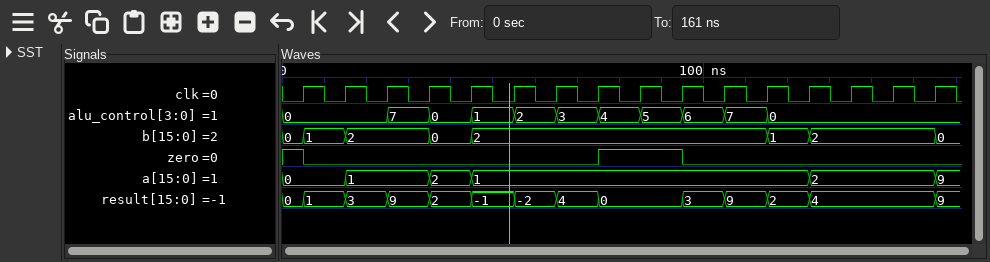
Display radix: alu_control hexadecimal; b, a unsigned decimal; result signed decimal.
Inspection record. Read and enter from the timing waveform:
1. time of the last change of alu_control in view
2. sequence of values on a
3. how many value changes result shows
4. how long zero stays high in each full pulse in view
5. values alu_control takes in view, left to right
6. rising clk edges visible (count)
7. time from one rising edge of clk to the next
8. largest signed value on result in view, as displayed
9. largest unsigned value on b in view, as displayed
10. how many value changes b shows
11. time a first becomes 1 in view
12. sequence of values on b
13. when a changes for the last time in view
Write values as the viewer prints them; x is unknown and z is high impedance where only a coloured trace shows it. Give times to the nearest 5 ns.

115 ns
0, 1, 2, 1, 2, 9
13
20 ns
0, 7, 0, 1, 2, 3, 4, 5, 6, 7, 0
16
10 ns
9
2
7
15 ns
0, 1, 2, 0, 2, 1, 2, 0
155 ns
